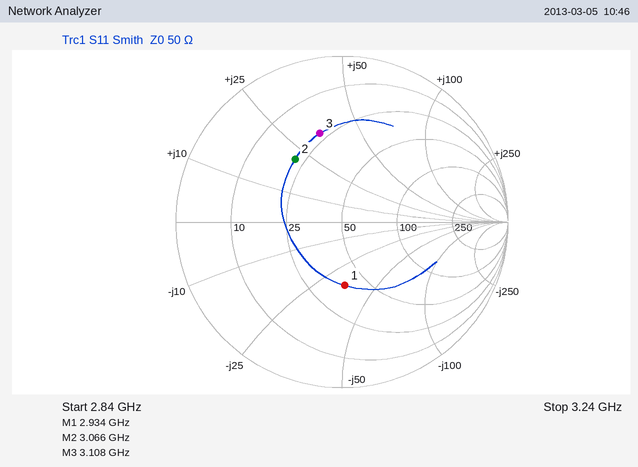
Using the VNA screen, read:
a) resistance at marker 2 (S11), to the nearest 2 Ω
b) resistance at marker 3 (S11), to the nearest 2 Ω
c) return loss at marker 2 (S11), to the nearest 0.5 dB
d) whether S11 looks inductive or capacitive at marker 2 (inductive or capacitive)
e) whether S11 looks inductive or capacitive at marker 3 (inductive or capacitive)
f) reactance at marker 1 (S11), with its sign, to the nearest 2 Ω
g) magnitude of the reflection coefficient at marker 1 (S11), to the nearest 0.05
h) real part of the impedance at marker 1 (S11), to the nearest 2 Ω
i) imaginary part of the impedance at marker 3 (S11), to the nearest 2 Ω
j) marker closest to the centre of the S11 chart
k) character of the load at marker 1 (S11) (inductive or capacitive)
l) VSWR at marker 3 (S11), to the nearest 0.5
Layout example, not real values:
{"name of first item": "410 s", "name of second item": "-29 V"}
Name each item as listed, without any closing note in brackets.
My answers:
{"resistance at marker 2 (S11), to the nearest 2 Ω": "22 Ω", "resistance at marker 3 (S11), to the nearest 2 Ω": "22 Ω", "return loss at marker 2 (S11), to the nearest 0.5 dB": "6.5 dB", "whether S11 looks inductive or capacitive at marker 2": "inductive", "whether S11 looks inductive or capacitive at marker 3": "inductive", "reactance at marker 1 (S11), with its sign, to the nearest 2 Ω": "-34 Ω", "magnitude of the reflection coefficient at marker 1 (S11), to the nearest 0.05": "0.40", "real part of the impedance at marker 1 (S11), to the nearest 2 Ω": "38 Ω", "imaginary part of the impedance at marker 3 (S11), to the nearest 2 Ω": "+34 Ω", "marker closest to the centre of the S11 chart": "marker 1", "character of the load at marker 1 (S11)": "capacitive", "VSWR at marker 3 (S11), to the nearest 0.5": "3.5"}
